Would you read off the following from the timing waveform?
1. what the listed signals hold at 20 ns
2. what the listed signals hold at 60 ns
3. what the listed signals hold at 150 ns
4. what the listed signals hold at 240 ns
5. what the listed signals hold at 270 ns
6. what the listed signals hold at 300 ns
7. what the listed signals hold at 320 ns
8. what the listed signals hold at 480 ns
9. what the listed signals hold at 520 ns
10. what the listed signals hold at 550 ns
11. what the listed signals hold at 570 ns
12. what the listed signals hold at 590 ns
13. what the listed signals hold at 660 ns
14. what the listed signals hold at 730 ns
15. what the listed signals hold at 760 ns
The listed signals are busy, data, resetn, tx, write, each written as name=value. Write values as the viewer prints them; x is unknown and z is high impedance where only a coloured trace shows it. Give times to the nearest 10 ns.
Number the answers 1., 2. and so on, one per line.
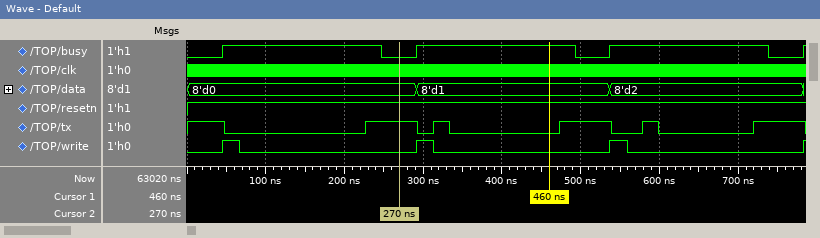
1. busy=0, data=8'd0, resetn=1, tx=1, write=0
2. busy=1, data=8'd0, resetn=1, tx=0, write=1
3. busy=1, data=8'd0, resetn=1, tx=0, write=0
4. busy=1, data=8'd0, resetn=1, tx=1, write=0
5. busy=0, data=8'd0, resetn=1, tx=1, write=0
6. busy=1, data=8'd1, resetn=1, tx=0, write=1
7. busy=1, data=8'd1, resetn=1, tx=1, write=0
8. busy=1, data=8'd1, resetn=1, tx=1, write=0
9. busy=0, data=8'd1, resetn=1, tx=1, write=0
10. busy=1, data=8'd2, resetn=1, tx=0, write=1
11. busy=1, data=8'd2, resetn=1, tx=0, write=0
12. busy=1, data=8'd2, resetn=1, tx=1, write=0
13. busy=1, data=8'd2, resetn=1, tx=0, write=0
14. busy=1, data=8'd2, resetn=1, tx=1, write=0
15. busy=0, data=8'd2, resetn=1, tx=1, write=0
